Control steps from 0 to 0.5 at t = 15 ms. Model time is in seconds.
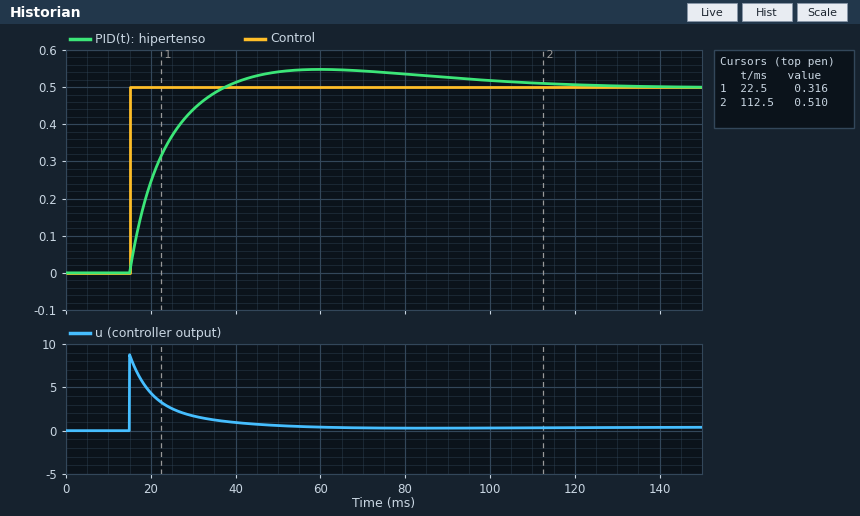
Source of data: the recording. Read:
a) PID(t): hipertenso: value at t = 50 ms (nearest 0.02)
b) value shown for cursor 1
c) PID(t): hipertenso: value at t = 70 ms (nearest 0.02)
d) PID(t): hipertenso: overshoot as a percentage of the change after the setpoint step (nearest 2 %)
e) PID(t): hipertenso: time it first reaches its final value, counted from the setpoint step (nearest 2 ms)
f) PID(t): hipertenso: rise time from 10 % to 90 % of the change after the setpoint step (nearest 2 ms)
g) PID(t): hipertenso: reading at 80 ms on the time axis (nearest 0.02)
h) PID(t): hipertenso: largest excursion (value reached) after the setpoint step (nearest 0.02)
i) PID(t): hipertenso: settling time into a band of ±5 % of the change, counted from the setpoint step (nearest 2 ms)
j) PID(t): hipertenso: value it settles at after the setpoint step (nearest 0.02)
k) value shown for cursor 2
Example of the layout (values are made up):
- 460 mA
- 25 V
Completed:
- 0.54
- 0.316
- 0.54
- 10 %
- 22 ms
- 16 ms
- 0.54
- 0.54
- 76 ms
- 0.50
- 0.510
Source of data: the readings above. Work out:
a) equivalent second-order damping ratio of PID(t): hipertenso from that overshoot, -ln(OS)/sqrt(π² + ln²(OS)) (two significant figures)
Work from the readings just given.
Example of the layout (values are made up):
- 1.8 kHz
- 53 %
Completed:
- 0.59
